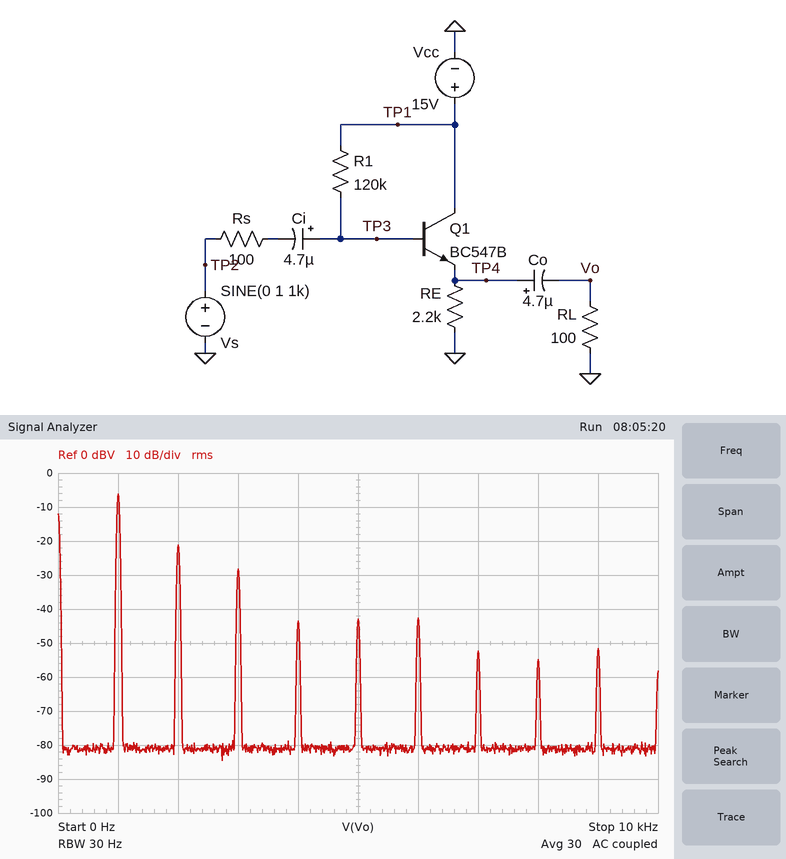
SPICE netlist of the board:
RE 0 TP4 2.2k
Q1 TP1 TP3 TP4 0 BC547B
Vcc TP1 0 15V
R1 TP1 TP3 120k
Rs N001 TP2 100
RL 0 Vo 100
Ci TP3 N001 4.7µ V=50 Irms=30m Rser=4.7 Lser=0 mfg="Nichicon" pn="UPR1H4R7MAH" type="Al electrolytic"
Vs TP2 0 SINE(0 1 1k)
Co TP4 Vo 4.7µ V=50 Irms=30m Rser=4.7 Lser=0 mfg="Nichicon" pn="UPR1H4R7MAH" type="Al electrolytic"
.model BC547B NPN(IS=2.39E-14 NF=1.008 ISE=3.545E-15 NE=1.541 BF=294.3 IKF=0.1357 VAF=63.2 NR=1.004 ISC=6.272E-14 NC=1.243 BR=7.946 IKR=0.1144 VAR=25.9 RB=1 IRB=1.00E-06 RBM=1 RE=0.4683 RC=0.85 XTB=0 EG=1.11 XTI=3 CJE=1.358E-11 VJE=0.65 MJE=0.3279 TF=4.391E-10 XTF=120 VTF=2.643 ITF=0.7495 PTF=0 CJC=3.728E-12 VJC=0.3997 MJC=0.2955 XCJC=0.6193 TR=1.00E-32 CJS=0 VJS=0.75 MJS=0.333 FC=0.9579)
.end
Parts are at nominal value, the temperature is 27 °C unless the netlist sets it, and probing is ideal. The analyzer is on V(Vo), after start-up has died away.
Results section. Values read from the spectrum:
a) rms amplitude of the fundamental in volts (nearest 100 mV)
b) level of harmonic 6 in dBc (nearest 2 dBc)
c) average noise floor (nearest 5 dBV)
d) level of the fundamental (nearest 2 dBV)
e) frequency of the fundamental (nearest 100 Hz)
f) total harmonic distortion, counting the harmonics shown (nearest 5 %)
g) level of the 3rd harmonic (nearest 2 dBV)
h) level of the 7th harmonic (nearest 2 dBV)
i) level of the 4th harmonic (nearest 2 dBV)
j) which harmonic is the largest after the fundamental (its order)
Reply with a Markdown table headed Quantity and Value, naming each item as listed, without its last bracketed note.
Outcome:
| Quantity | Value |
|---|---|
| rms amplitude of the fundamental in volts | 500 mV |
| level of harmonic 6 in dBc | -36 dBc |
| average noise floor | -80 dBV |
| level of the fundamental | -6 dBV |
| frequency of the fundamental | 1.0 kHz |
| total harmonic distortion, counting the harmonics shown | 20 % |
| level of the 3rd harmonic | -28 dBV |
| level of the 7th harmonic | -52 dBV |
| level of the 4th harmonic | -44 dBV |
| which harmonic is the largest after the fundamental | 2 |
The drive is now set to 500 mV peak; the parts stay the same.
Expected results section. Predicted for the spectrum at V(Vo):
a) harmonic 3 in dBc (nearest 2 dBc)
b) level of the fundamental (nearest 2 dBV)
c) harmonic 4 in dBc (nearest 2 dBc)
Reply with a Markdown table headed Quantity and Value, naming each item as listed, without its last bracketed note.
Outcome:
| Quantity | Value |
|---|---|
| harmonic 3 in dBc | -48 dBc |
| level of the fundamental | -10 dBV |
| harmonic 4 in dBc | -56 dBc |
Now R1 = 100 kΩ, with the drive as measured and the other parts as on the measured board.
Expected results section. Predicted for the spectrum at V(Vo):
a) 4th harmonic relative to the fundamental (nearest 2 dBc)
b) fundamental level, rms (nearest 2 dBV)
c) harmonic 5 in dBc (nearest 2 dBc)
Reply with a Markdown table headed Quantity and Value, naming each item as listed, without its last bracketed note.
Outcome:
| Quantity | Value |
|---|---|
| 4th harmonic relative to the fundamental | -36 dBc |
| fundamental level, rms | -6 dBV |
| harmonic 5 in dBc | -38 dBc |
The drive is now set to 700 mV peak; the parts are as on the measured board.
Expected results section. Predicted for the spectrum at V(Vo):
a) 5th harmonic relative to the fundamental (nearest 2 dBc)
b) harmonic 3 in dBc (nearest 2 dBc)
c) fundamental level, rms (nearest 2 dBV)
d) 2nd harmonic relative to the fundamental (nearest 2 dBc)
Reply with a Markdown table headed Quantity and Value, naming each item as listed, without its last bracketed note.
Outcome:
| Quantity | Value |
|---|---|
| 5th harmonic relative to the fundamental | -42 dBc |
| harmonic 3 in dBc | -32 dBc |
| fundamental level, rms | -8 dBV |
| 2nd harmonic relative to the fundamental | -26 dBc |
